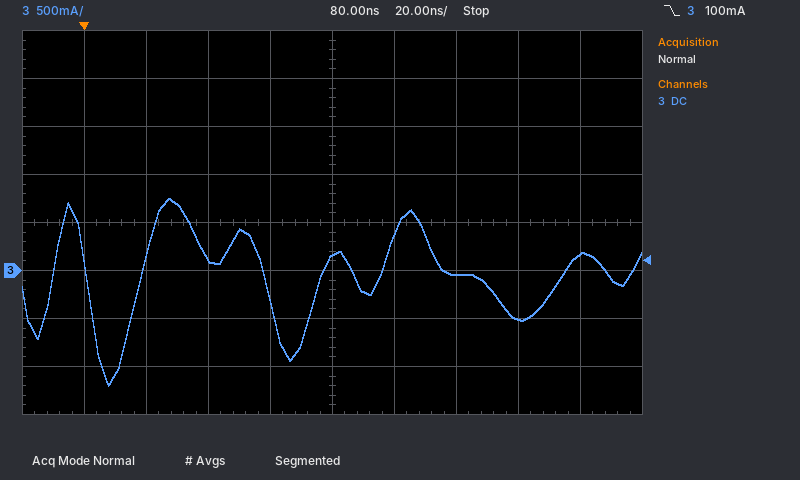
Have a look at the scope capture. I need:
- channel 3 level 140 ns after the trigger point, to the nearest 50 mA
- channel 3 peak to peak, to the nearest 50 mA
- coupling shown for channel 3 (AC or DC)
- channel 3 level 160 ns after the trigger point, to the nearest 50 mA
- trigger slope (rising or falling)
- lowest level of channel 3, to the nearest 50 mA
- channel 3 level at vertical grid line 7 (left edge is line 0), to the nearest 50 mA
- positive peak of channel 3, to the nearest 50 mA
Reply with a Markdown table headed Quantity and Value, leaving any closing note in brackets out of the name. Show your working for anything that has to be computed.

| Quantity | Value |
|---|---|
| channel 3 level 140 ns after the trigger point, to the nearest 50 mA | -500 mA |
| channel 3 peak to peak, to the nearest 50 mA | 750 mA − (-1.20 A) = 1.95 A |
| coupling shown for channel 3 | DC |
| channel 3 level 160 ns after the trigger point, to the nearest 50 mA | 150 mA |
| trigger slope | falling |
| lowest level of channel 3, to the nearest 50 mA | -1.20 A |
| channel 3 level at vertical grid line 7 (left edge is line 0), to the nearest 50 mA | -50 mA |
| positive peak of channel 3, to the nearest 50 mA | 750 mA |
